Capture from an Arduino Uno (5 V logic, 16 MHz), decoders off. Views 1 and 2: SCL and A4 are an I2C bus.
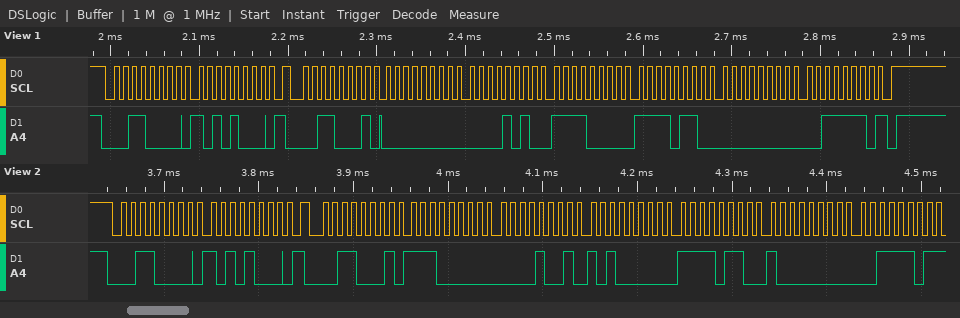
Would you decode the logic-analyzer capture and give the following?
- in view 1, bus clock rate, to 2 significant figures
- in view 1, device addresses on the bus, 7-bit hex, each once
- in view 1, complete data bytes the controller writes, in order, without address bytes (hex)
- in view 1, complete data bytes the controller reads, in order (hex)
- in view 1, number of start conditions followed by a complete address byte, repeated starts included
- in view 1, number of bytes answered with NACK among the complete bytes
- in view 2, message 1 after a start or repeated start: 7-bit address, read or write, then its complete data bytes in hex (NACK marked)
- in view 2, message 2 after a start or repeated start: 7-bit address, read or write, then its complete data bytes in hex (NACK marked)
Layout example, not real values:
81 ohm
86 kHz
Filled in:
100 kHz
0x18
A8
00 0A F0 F6 00 3E
2
1
0x18 write: A8
0x18 read: E0 09 A0 F6 80 3D NACK
